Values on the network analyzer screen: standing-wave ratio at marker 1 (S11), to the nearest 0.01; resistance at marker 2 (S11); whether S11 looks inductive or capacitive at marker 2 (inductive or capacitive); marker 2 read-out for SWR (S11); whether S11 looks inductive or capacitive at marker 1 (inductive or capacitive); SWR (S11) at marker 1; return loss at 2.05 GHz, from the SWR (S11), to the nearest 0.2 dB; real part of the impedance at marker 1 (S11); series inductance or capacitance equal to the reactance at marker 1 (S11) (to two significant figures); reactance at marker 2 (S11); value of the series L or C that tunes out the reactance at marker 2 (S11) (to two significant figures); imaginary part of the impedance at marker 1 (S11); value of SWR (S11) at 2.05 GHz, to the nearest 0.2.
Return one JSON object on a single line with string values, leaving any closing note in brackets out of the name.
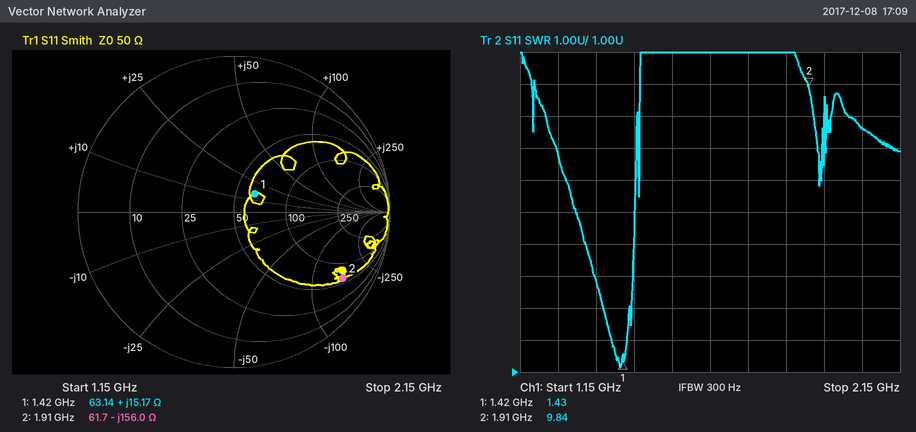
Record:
{"standing-wave ratio at marker 1 (S11), to the nearest 0.01": "1.43", "resistance at marker 2": "61.7 Ω", "whether S11 looks inductive or capacitive at marker 2": "capacitive", "marker 2 read-out for SWR": "9.84", "whether S11 looks inductive or capacitive at marker 1": "inductive", "SWR (S11) at marker 1": "1.43", "return loss at 2.05 GHz, from the SWR (S11), to the nearest 0.2 dB": "2.0 dB", "real part of the impedance at marker 1": "63.14 Ω", "series inductance or capacitance equal to the reactance at marker 1 (S11)": "1.7 nH", "reactance at marker 2": "-156.0 Ω", "value of the series L or C that tunes out the reactance at marker 2 (S11)": "13 nH", "imaginary part of the impedance at marker 1": "+15.17 Ω", "value of SWR (S11) at 2.05 GHz, to the nearest 0.2": "8.6"}
